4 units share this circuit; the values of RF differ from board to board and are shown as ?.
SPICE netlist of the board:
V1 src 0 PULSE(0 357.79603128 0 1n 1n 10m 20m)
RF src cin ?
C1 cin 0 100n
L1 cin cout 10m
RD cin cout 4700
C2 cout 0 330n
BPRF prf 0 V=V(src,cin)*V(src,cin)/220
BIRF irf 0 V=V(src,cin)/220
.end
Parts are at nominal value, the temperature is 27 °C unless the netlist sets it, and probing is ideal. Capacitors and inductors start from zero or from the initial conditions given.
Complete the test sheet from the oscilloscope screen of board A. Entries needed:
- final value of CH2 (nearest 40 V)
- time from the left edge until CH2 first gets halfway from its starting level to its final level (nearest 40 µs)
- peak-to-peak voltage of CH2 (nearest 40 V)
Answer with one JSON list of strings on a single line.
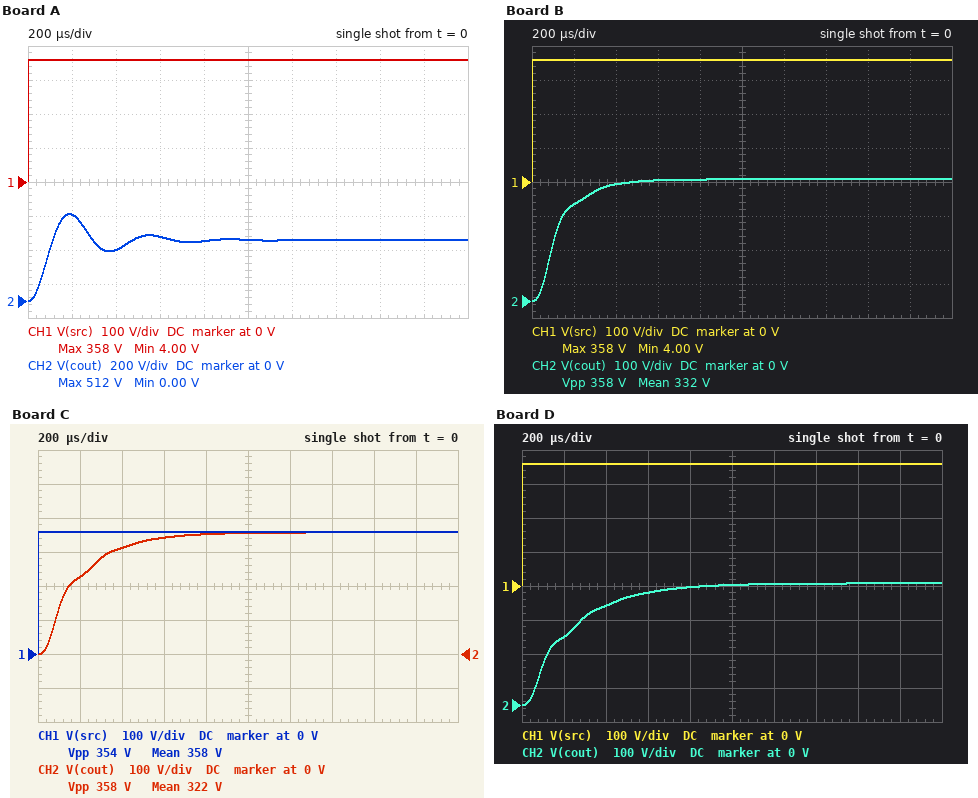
["360 V", "80 µs", "520 V"]
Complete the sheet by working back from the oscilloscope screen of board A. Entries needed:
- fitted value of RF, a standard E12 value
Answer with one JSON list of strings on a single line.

["82 Ω"]
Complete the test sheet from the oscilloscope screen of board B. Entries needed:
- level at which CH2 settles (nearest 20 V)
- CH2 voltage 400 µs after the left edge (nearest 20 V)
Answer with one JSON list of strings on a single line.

["360 V", "340 V"]
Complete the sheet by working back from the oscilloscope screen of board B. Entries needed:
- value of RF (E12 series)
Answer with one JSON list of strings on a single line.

["330 Ω"]
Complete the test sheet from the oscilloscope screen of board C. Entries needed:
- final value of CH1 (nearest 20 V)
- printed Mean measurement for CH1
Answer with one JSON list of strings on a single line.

["360 V", "358 V"]
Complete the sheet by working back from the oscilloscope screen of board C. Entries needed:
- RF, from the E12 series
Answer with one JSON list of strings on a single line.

["470 Ω"]
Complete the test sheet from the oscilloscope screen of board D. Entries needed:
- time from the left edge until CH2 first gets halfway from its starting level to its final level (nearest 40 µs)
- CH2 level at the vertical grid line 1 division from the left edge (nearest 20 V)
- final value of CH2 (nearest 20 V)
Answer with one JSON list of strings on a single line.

["160 µs", "200 V", "360 V"]
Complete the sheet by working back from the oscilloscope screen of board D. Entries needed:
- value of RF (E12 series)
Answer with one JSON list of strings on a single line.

["560 Ω"]
